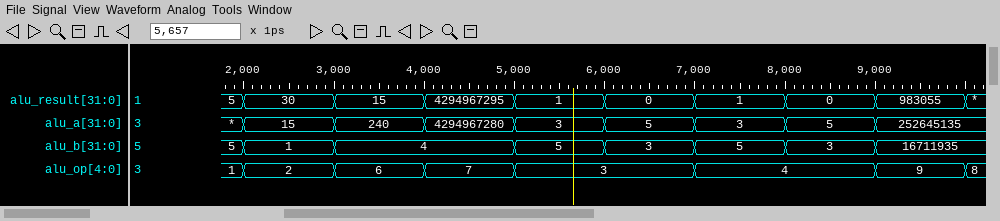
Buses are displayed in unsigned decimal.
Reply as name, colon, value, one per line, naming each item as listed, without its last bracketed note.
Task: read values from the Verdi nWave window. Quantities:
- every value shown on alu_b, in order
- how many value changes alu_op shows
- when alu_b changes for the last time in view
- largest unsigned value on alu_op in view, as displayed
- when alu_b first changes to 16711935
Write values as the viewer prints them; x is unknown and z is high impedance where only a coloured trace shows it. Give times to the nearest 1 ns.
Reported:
every value shown on alu_b, in order: 5, 1, 4, 5, 3, 5, 3, 16711935
how many value changes alu_op shows: 7
when alu_b changes for the last time in view: 9 ns
largest unsigned value on alu_op in view, as displayed: 9
when alu_b first changes to 16711935: 9 ns
